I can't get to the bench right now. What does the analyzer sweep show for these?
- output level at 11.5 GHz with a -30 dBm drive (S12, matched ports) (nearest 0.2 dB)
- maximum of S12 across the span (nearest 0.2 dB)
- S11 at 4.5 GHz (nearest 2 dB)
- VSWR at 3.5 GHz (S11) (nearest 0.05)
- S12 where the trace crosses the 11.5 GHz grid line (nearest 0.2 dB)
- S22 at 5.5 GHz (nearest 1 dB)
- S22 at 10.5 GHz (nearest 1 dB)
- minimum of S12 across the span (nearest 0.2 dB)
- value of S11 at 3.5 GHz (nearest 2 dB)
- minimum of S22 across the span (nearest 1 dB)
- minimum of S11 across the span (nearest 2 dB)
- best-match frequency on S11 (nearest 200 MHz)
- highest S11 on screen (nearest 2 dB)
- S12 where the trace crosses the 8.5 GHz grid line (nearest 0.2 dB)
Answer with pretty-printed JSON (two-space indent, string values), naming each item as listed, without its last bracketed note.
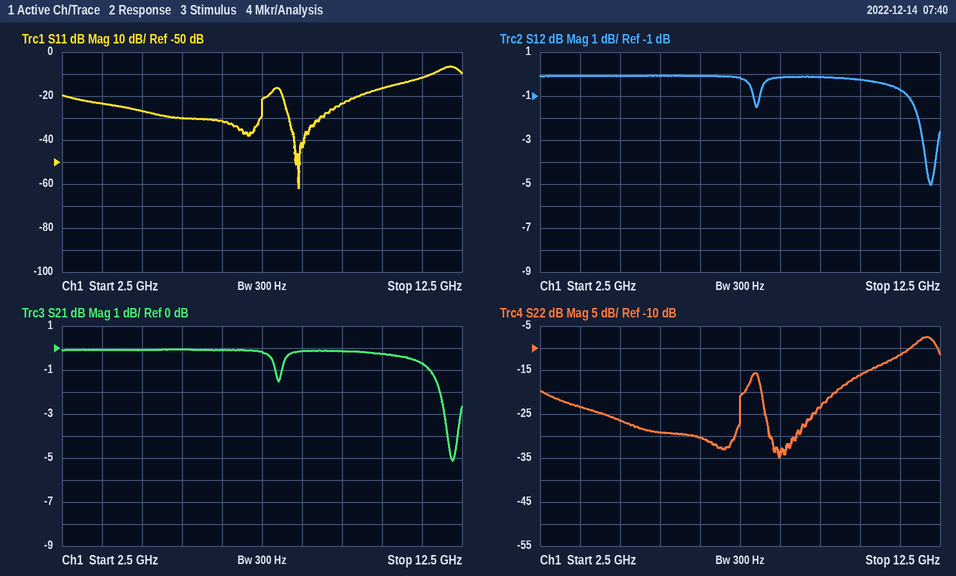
{
  "output level at 11.5 GHz with a -30 dBm drive (S12, matched ports)": "-30.8 dBm",
  "maximum of S12 across the span": "0.0 dB",
  "S11 at 4.5 GHz": "-26 dB",
  "VSWR at 3.5 GHz (S11)": "1.15",
  "S12 where the trace crosses the 11.5 GHz grid line": "-0.8 dB",
  "S22 at 5.5 GHz": "-29 dB",
  "S22 at 10.5 GHz": "-16 dB",
  "minimum of S12 across the span": "-5.0 dB",
  "value of S11 at 3.5 GHz": "-24 dB",
  "minimum of S22 across the span": "-35 dB",
  "minimum of S11 across the span": "-62 dB",
  "best-match frequency on S11": "8.4 GHz",
  "highest S11 on screen": "-6 dB",
  "S12 where the trace crosses the 8.5 GHz grid line": "-0.2 dB"
}
